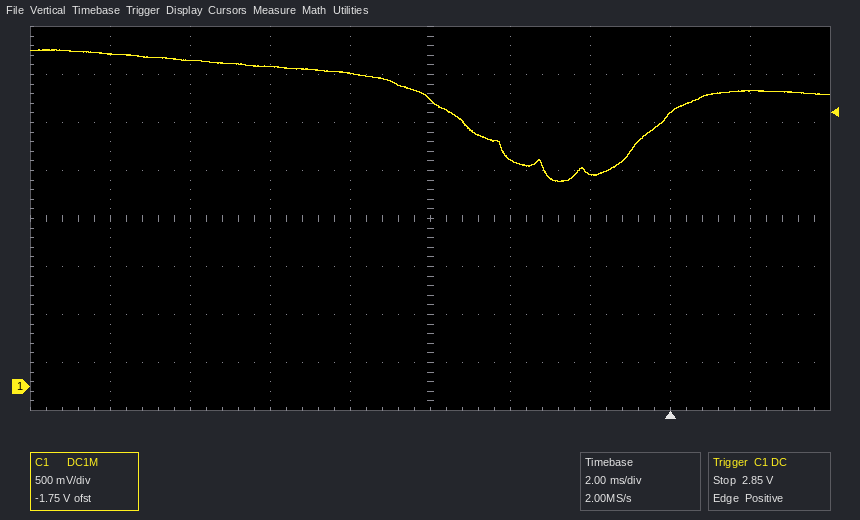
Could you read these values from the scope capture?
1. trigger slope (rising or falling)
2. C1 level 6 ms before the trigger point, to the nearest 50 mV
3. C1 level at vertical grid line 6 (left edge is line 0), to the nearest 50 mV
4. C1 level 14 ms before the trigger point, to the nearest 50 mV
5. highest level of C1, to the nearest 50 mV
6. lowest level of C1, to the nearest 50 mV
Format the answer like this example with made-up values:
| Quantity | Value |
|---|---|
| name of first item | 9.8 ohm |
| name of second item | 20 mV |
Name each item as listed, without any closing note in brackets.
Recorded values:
| Quantity | Value |
|---|---|
| trigger slope | rising |
| C1 level 6 ms before the trigger point, to the nearest 50 mV | 3.00 V |
| C1 level at vertical grid line 6 (left edge is line 0), to the nearest 50 mV | 2.35 V |
| C1 level 14 ms before the trigger point, to the nearest 50 mV | 3.45 V |
| highest level of C1, to the nearest 50 mV | 3.50 V |
| lowest level of C1, to the nearest 50 mV | 2.15 V |
